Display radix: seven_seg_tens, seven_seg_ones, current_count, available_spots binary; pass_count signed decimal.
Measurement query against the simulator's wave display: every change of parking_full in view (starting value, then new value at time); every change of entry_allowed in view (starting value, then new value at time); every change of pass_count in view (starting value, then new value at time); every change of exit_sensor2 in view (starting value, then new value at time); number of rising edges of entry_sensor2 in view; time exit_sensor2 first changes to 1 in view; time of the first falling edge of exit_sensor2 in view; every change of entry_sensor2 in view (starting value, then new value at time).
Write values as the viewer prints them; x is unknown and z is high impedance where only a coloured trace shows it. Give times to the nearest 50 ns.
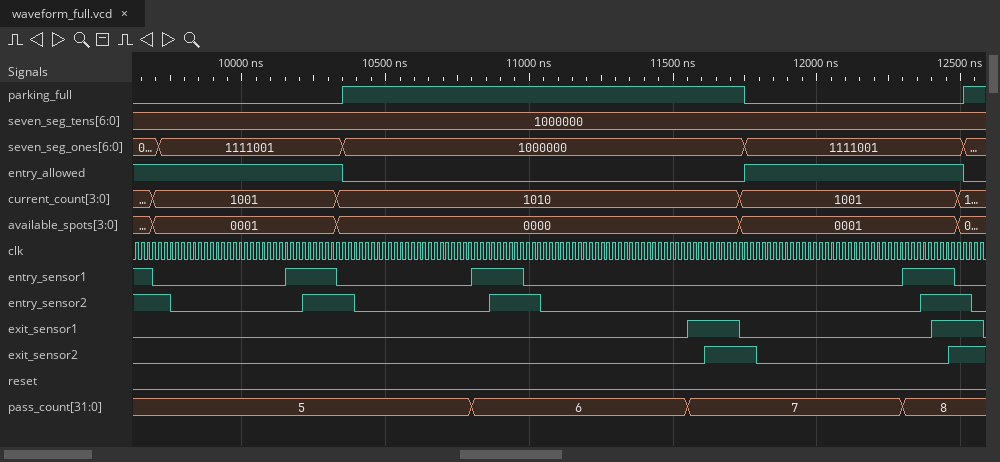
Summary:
0, 1 at 10350 ns, 0 at 11750 ns, 1 at 12500 ns
1, 0 at 10350 ns, 1 at 11750 ns, 0 at 12500 ns
5, 6 at 10800 ns, 7 at 11550 ns, 8 at 12300 ns
0, 1 at 11600 ns, 0 at 11800 ns, 1 at 12450 ns
3
11600 ns
11800 ns
1, 0 at 9750 ns, 1 at 10200 ns, 0 at 10400 ns, 1 at 10850 ns, 0 at 11050 ns, 1 at 12350 ns, 0 at 12550 ns
